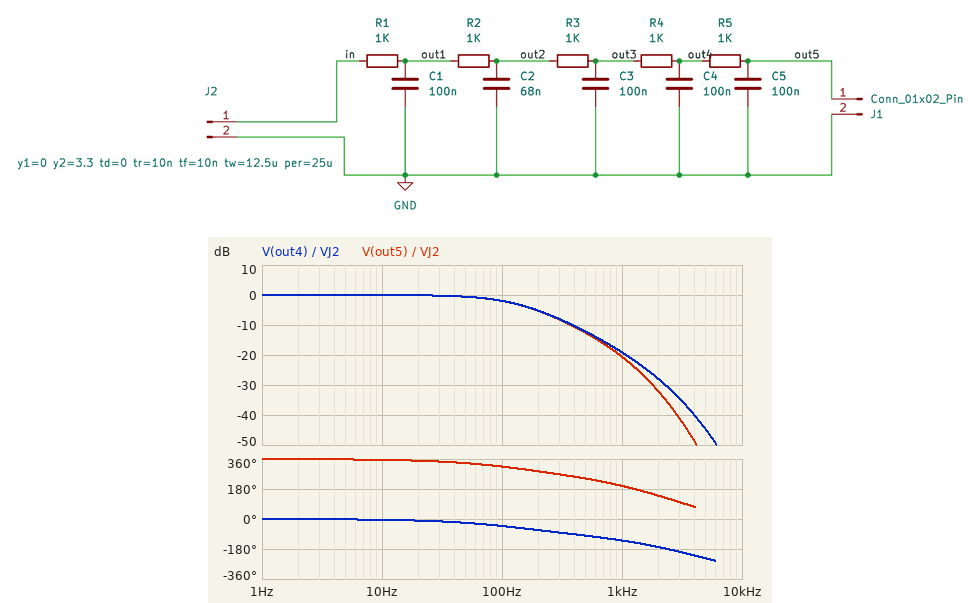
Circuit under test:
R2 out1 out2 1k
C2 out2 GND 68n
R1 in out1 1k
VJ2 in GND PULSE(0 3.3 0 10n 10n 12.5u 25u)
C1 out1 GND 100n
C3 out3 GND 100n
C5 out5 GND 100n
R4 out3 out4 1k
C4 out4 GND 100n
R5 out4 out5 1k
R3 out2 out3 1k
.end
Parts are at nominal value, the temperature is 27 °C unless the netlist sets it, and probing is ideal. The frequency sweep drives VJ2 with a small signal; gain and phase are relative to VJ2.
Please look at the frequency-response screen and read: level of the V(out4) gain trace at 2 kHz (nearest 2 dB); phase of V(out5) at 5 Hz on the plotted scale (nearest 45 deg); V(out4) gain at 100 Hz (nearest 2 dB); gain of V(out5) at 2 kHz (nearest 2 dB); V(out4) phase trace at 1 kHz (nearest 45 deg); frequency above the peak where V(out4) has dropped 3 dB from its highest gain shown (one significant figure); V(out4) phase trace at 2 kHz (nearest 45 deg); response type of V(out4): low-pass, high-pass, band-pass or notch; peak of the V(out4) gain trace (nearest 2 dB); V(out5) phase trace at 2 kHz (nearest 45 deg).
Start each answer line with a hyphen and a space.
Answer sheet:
- -28 dB
- 360 deg
- -2 dB
- -32 dB
- -135 deg
- 100 Hz
- -180 deg
- low-pass
- 0 dB
- 135 deg
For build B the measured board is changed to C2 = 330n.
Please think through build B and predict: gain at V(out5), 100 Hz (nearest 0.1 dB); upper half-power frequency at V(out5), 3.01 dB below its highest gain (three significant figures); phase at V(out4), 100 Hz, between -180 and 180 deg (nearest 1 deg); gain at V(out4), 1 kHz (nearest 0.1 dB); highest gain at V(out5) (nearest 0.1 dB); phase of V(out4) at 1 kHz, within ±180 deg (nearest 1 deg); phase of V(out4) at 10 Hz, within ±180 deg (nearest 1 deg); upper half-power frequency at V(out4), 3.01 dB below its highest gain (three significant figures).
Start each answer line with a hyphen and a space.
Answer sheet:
- -3.1 dB
- 98.5 Hz
- -55 deg
- -25.0 dB
- 0 dB
- -157 deg
- -7 deg
- 98.9 Hz
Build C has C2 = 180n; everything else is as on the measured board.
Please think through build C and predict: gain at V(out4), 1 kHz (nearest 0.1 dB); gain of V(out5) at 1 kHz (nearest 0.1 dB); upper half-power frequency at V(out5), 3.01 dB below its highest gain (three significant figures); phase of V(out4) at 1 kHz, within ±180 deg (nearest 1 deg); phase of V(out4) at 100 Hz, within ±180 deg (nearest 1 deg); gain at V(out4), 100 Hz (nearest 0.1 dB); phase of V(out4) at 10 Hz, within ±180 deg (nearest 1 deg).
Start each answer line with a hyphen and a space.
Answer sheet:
- -21.9 dB
- -23.3 dB
- 116 Hz
- -146 deg
- -48 deg
- -2.4 dB
- -6 deg
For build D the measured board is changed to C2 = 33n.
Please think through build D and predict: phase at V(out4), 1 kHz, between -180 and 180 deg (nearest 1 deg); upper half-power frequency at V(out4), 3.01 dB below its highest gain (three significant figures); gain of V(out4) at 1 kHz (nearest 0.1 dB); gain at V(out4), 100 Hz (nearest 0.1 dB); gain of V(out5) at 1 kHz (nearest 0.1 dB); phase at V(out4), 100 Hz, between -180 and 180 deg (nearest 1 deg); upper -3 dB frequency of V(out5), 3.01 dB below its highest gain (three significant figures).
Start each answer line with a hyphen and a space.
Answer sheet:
- -121 deg
- 138 Hz
- -18.3 dB
- -1.8 dB
- -19.8 dB
- -40 deg
- 137 Hz
